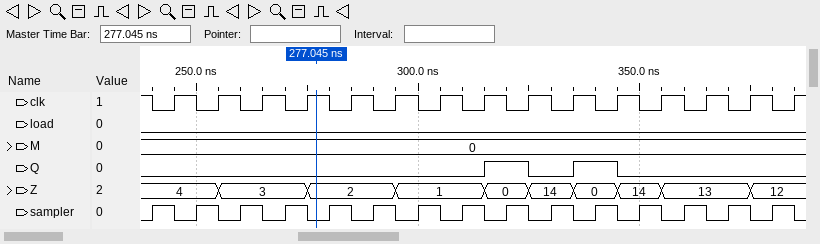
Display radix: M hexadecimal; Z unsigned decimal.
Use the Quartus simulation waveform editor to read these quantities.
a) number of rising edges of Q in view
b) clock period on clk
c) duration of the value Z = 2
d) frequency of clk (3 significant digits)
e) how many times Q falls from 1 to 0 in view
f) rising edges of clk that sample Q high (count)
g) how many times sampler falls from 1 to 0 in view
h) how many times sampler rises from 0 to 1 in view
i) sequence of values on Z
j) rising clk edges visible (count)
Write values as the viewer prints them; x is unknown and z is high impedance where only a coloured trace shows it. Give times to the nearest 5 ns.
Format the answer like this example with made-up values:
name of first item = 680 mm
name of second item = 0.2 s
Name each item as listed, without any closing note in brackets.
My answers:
number of rising edges of Q in view = 2
clock period on clk = 10 ns
duration of the value Z = 2 = 20 ns
frequency of clk = 100 MHz
how many times Q falls from 1 to 0 in view = 2
rising edges of clk that sample Q high = 2
how many times sampler falls from 1 to 0 in view = 15
how many times sampler rises from 0 to 1 in view = 15
sequence of values on Z = 4, 3, 2, 1, 0, 14, 0, 14, 13, 12
rising clk edges visible = 15
